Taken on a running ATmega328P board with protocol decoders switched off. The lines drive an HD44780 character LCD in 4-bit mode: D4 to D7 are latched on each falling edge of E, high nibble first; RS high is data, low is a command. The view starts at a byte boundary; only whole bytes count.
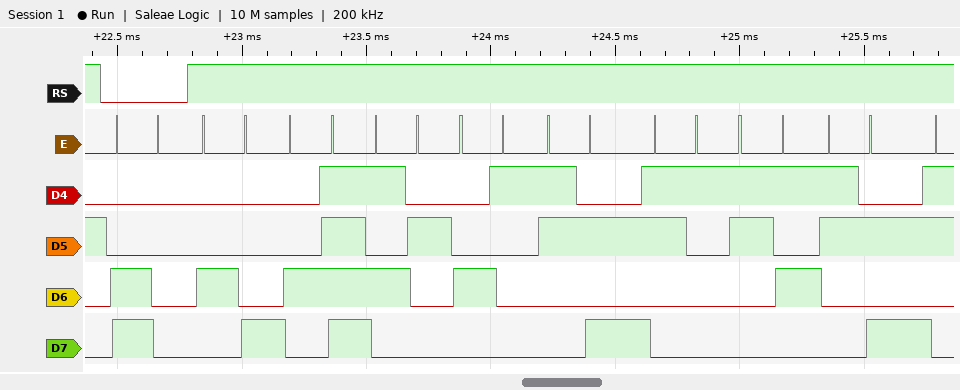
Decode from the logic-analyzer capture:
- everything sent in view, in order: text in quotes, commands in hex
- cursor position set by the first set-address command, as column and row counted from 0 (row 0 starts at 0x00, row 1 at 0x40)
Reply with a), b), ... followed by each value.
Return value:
a) 0xC0 "HORA:15:"
b) column 0, row 1
